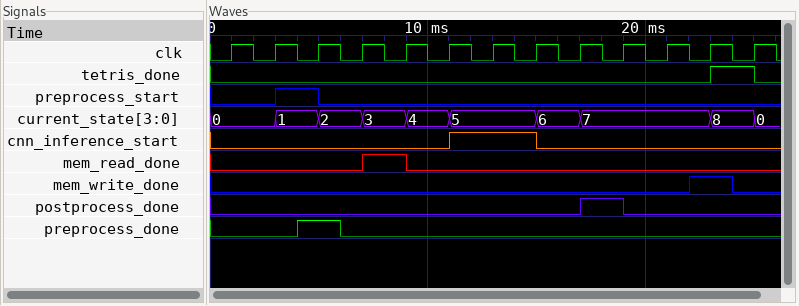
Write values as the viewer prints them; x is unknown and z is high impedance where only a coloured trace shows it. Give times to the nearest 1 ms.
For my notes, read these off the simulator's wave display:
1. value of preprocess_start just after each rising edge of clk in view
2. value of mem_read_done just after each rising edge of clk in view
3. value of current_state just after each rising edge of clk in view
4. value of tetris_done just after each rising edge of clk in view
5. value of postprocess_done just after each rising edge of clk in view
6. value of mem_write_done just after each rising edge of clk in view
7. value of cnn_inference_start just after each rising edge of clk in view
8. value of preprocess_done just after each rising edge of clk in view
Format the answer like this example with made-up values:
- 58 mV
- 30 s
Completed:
- 0 1 0 0 0 0 0 0 0 0 0 0 0
- 0 0 0 1 0 0 0 0 0 0 0 0 0
- 0, 1, 2, 3, 4, 5, 5, 6, 7, 7, 7, 8, 0
- 0 0 0 0 0 0 0 0 0 0 0 1 0
- 0 0 0 0 0 0 0 0 1 0 0 0 0
- 0 0 0 0 0 0 0 0 0 0 0 1 0
- 0 0 0 0 0 1 1 0 0 0 0 0 0
- 0 0 1 0 0 0 0 0 0 0 0 0 0
